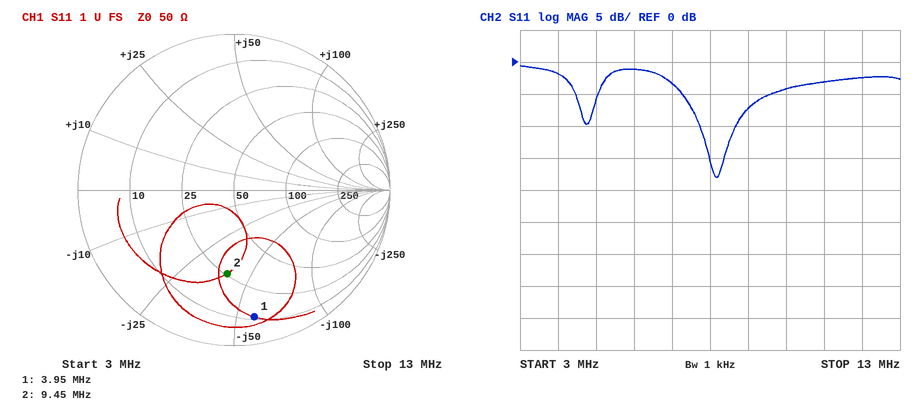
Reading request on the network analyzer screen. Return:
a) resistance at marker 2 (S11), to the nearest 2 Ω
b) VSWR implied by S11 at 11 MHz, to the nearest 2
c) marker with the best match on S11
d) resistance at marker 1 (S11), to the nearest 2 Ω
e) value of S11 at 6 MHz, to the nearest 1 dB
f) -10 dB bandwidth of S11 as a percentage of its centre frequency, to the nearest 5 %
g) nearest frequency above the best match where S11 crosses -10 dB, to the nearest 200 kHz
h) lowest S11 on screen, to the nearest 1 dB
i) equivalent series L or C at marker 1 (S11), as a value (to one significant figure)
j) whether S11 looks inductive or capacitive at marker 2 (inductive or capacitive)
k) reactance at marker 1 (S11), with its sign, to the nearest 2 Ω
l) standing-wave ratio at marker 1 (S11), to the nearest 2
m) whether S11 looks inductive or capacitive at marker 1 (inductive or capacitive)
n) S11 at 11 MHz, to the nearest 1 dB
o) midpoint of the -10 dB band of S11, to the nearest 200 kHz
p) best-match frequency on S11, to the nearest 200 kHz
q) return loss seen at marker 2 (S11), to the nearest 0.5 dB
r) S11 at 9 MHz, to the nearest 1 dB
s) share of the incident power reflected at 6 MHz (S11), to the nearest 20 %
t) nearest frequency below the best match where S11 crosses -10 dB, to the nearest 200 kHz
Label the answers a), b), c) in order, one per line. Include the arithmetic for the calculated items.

a) 26 Ω
b) |Γ| = 10^(-3/20) = 0.7079; VSWR = (1 + 0.7079)/(1 − 0.7079) ≈ 6
c) marker 2
d) 12 Ω
e) -1 dB
f) 800 kHz / 8.2 MHz ≈ 10 %
g) 8.6 MHz
h) -18 dB
i) C = 1/(2π × 3.95 MHz × 58 Ω) ≈ 695 pF, so 700 pF to one significant figure
j) capacitive
k) -58 Ω
l) 10
m) capacitive
n) -3 dB
o) 8.2 MHz
p) 8.2 MHz
q) 5.5 dB
r) -7 dB
s) 10^(-1/10) ≈ 79.4 %, so 80 % to the nearest 20 %
t) 7.8 MHz
